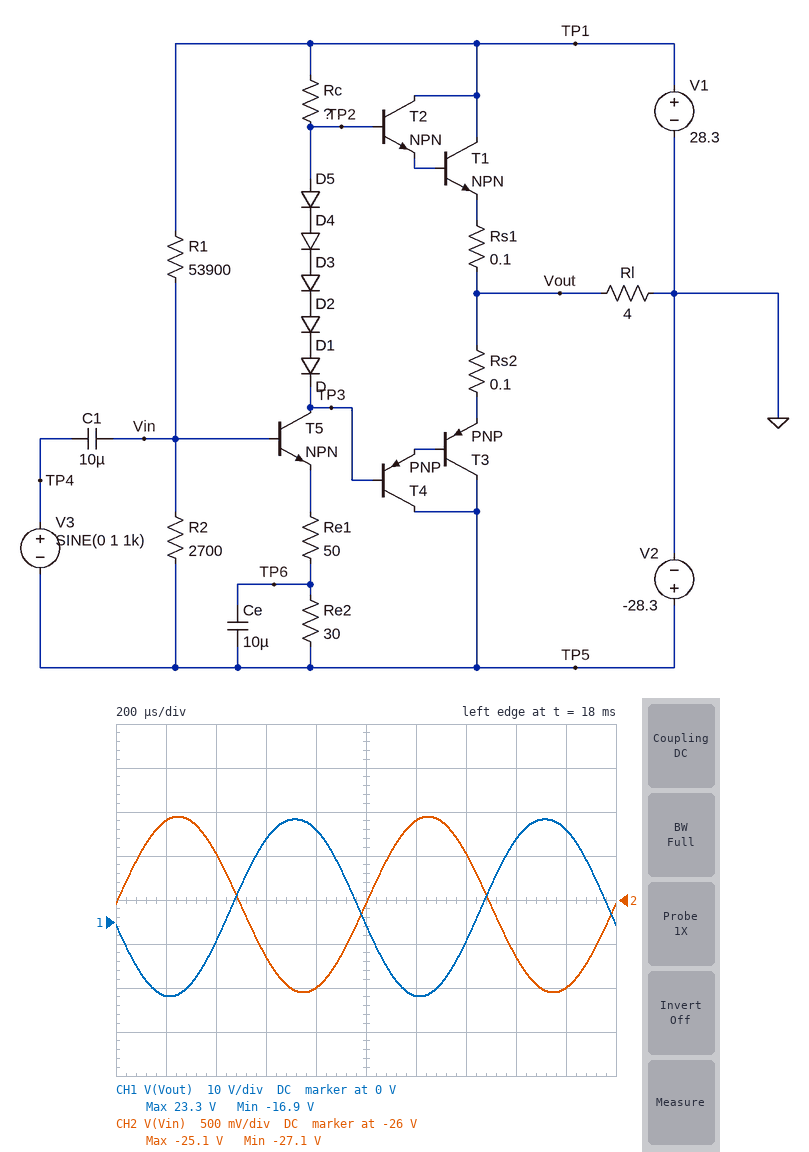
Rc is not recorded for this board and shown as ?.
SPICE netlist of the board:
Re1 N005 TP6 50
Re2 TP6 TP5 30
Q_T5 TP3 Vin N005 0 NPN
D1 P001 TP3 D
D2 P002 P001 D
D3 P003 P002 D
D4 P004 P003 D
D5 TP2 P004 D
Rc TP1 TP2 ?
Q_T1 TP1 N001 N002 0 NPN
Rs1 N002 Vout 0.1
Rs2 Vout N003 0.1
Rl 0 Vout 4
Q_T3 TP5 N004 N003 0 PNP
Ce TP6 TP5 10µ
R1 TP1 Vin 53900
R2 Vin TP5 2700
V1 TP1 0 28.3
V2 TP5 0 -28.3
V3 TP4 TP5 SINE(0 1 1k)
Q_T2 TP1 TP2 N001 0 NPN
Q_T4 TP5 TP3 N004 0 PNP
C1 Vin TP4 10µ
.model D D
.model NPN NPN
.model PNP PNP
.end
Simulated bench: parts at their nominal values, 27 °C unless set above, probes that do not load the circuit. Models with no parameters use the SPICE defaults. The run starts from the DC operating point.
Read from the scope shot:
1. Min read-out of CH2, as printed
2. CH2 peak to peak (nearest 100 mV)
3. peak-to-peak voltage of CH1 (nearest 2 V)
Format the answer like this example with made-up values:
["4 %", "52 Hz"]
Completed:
["-27.1 V", "2.0 V", "40 V"]
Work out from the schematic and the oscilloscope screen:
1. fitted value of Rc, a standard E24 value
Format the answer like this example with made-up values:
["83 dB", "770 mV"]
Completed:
["1.3 kΩ"]
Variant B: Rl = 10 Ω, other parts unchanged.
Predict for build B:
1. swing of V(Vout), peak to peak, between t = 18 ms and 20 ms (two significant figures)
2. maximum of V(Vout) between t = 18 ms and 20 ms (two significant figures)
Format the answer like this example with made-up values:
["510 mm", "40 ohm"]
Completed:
["42 V", "24 V"]
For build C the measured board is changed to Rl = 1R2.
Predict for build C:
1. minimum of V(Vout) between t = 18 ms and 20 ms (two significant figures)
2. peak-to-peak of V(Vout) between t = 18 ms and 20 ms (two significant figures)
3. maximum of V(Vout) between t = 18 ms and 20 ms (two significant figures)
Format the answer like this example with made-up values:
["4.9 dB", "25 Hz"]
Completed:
["-15 V", "36 V", "21 V"]
